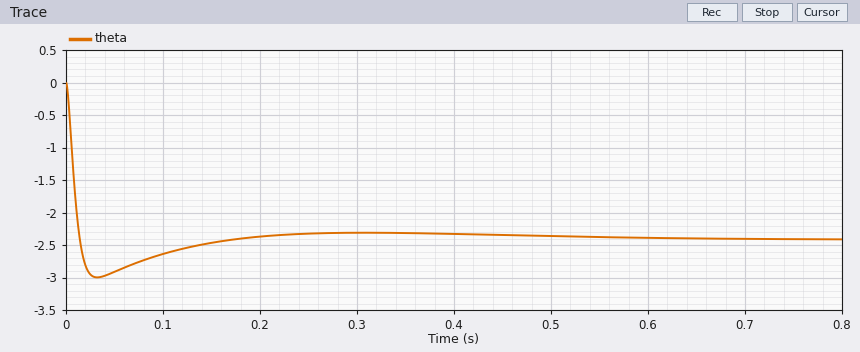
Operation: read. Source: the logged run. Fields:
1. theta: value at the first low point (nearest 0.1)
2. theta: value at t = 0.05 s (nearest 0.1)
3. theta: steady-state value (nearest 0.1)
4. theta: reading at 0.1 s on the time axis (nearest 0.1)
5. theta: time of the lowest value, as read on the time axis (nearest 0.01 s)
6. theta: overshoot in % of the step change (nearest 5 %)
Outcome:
-3.0
-2.9
-2.4
-2.6
0.03 s
25 %
